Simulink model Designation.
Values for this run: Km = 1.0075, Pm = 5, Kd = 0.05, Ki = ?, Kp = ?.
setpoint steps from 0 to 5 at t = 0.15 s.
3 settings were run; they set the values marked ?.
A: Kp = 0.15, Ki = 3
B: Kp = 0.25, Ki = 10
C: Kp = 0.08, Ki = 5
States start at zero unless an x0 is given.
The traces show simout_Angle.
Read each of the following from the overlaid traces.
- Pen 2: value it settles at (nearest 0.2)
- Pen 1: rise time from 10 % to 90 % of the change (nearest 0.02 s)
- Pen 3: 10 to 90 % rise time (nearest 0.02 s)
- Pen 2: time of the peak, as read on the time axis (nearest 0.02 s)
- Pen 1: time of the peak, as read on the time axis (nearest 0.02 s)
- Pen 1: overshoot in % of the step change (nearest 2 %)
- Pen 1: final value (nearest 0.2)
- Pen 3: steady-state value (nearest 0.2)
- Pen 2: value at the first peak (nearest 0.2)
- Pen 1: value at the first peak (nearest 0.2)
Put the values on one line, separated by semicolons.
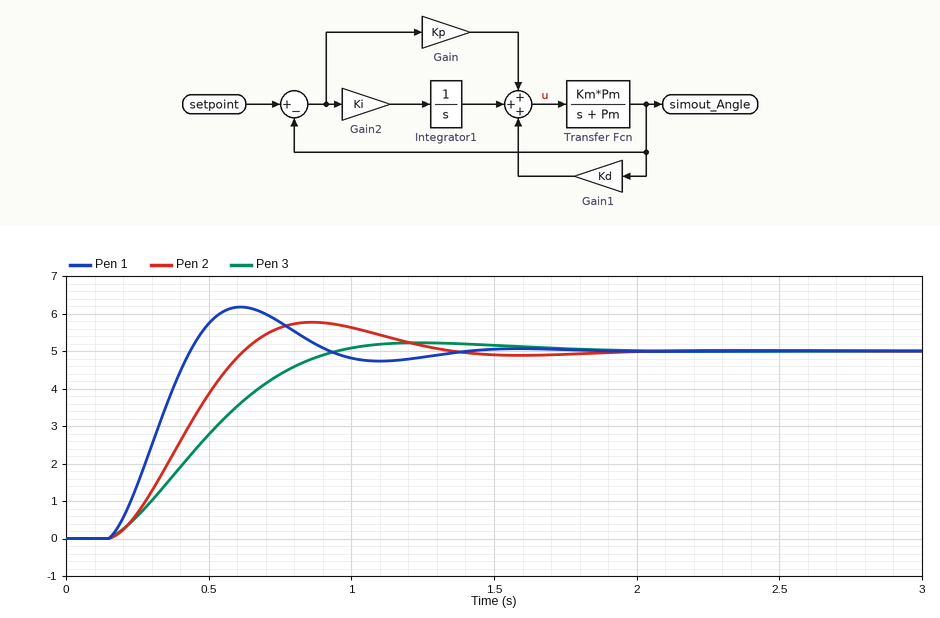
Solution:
5.0; 0.20 s; 0.54 s; 0.86 s; 0.62 s; 24 %; 5.0; 5.0; 5.8; 6.2
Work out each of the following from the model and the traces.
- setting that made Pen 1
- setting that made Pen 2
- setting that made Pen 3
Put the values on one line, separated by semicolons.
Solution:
B; C; A
